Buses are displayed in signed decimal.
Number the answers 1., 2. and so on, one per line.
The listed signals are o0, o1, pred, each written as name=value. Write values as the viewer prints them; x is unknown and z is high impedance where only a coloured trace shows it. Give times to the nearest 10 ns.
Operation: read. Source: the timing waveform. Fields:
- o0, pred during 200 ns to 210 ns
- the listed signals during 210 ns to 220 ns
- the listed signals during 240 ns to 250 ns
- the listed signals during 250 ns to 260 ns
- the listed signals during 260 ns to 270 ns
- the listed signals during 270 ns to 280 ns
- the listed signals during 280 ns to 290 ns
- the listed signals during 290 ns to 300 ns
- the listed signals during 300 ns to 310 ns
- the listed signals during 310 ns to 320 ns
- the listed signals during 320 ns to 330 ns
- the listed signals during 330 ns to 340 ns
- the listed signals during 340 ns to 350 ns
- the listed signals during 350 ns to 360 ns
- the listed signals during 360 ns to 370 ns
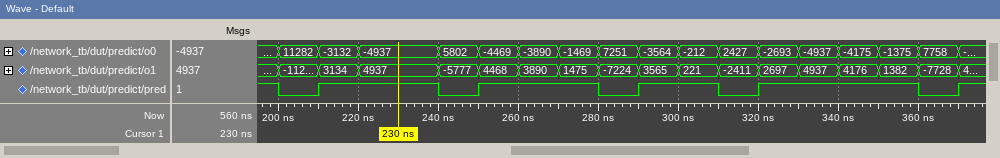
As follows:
1. o0=11282, pred=0
2. o0=-3132, o1=3134, pred=1
3. o0=5802, o1=-5777, pred=0
4. o0=-4469, o1=4468, pred=1
5. o0=-3890, o1=3890, pred=1
6. o0=-1469, o1=1475, pred=1
7. o0=7251, o1=-7224, pred=0
8. o0=-3564, o1=3565, pred=1
9. o0=-212, o1=221, pred=1
10. o0=2427, o1=-2411, pred=0
11. o0=-2693, o1=2697, pred=1
12. o0=-4937, o1=4937, pred=1
13. o0=-4175, o1=4176, pred=1
14. o0=-1375, o1=1382, pred=1
15. o0=7758, o1=-7728, pred=0
